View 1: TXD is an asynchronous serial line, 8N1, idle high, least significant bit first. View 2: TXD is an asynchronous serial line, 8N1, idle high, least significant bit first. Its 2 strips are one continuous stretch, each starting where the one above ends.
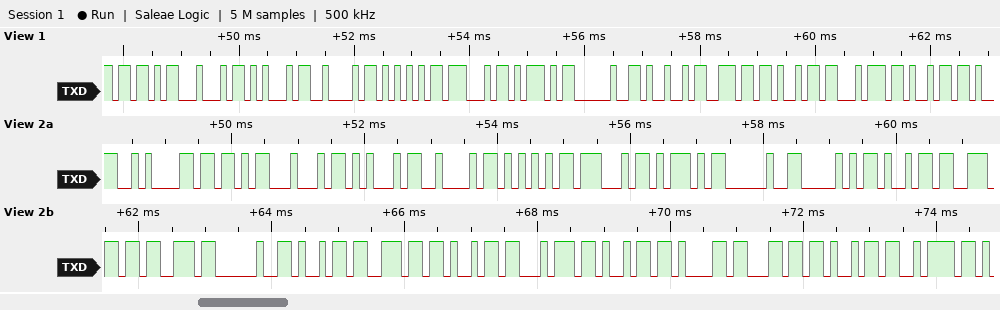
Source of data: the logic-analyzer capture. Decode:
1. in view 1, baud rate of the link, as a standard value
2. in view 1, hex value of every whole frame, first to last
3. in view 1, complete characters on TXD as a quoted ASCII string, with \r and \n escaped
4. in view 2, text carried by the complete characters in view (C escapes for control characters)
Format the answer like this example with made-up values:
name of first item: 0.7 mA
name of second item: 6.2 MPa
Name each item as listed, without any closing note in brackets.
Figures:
in view 1, baud rate of the link, as a standard value: 9600 baud
in view 1, hex value of every whole frame, first to last: 0x5B 0x44 0x45 0x42 0x55 0x47 0x5D 0x20 0x49 0x6E 0x69 0x74 0x69
in view 1, complete characters on TXD as a quoted ASCII string, with \r and \n escaped: "[DEBUG] Initi"
in view 2, text carried by the complete characters in view: "\n[DEBUG] Pins initializ"
